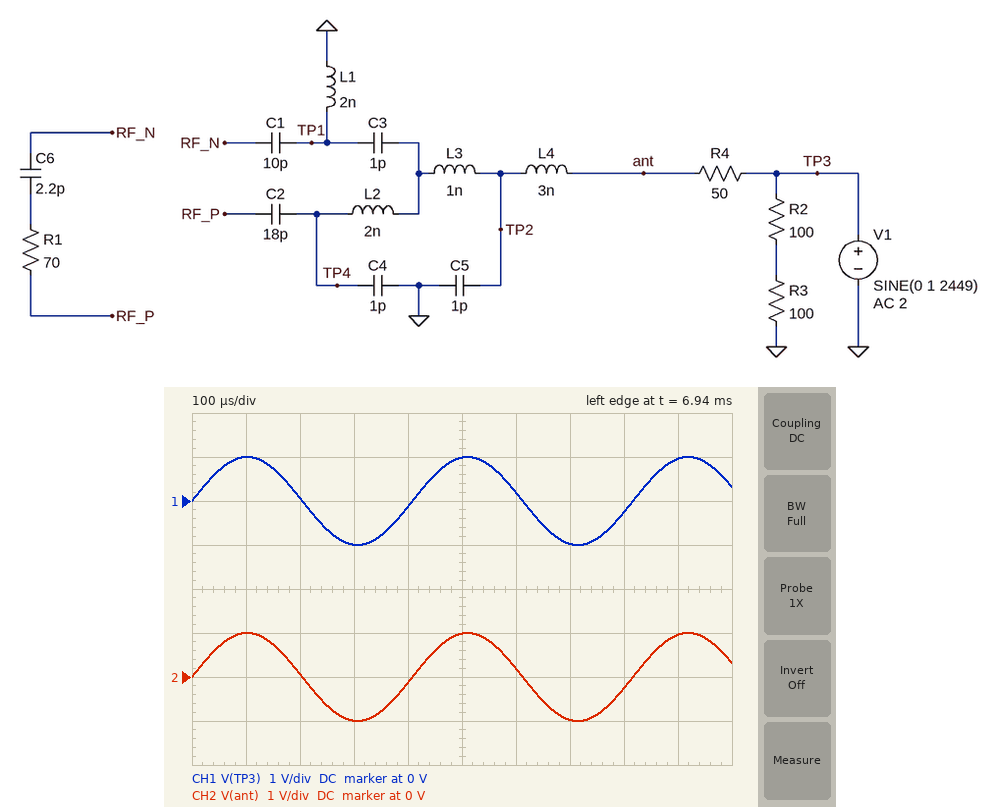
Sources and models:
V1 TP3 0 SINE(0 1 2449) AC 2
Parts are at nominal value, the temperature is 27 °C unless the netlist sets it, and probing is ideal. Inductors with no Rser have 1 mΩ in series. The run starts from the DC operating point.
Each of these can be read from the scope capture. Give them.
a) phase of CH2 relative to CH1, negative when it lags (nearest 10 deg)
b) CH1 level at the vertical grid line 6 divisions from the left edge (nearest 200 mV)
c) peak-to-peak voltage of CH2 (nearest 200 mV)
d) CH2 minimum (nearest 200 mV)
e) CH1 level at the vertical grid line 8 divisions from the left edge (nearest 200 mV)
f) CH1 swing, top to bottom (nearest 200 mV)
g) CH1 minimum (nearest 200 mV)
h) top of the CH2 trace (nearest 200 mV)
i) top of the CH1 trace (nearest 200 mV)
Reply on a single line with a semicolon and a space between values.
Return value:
0 deg; 200 mV; 2.0 V; -1.0 V; -200 mV; 2.0 V; -1.0 V; 1.0 V; 1.0 V
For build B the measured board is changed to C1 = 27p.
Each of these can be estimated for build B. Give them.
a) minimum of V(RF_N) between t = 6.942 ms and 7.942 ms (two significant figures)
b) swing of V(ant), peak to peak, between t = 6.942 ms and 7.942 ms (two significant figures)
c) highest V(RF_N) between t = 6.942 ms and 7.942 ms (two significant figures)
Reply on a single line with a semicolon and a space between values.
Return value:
-68 mV; 2.0 V; 68 mV
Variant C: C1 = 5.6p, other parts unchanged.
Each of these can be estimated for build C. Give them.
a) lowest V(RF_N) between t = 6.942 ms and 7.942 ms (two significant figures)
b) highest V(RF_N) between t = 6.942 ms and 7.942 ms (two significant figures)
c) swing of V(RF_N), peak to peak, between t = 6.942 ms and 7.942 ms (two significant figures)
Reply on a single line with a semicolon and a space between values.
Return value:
-260 mV; 260 mV; 520 mV
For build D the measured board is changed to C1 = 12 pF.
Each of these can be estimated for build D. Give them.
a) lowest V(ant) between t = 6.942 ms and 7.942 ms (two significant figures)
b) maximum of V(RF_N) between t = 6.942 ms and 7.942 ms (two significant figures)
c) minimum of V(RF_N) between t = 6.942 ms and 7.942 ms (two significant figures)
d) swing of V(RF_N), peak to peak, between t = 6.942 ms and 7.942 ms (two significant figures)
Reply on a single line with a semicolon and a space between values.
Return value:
-1.0 V; 140 mV; -140 mV; 280 mV
